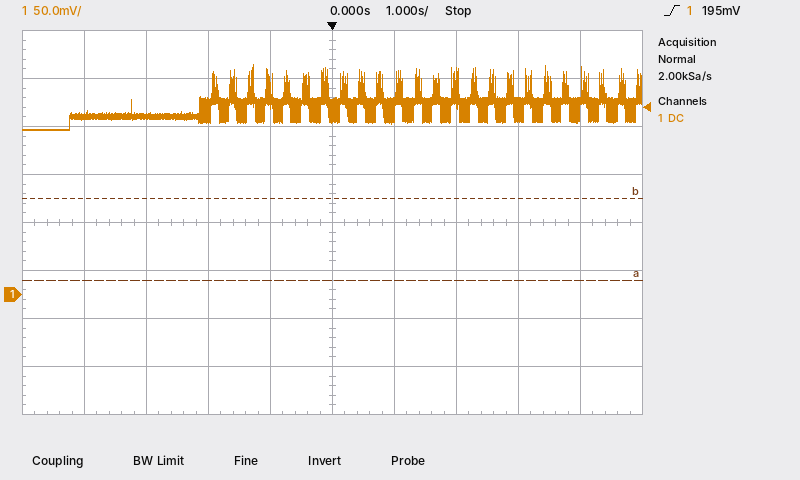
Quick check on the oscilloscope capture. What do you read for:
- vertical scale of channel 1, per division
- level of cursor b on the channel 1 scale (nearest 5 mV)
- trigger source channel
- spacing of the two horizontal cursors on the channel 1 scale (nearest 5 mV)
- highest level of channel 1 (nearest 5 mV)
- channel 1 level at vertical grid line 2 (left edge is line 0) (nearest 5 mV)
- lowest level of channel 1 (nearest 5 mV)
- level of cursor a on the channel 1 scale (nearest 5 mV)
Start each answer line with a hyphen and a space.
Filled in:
- 50 mV
- 100 mV
- channel 1
- 85 mV
- 240 mV
- 185 mV
- 170 mV
- 15 mV
